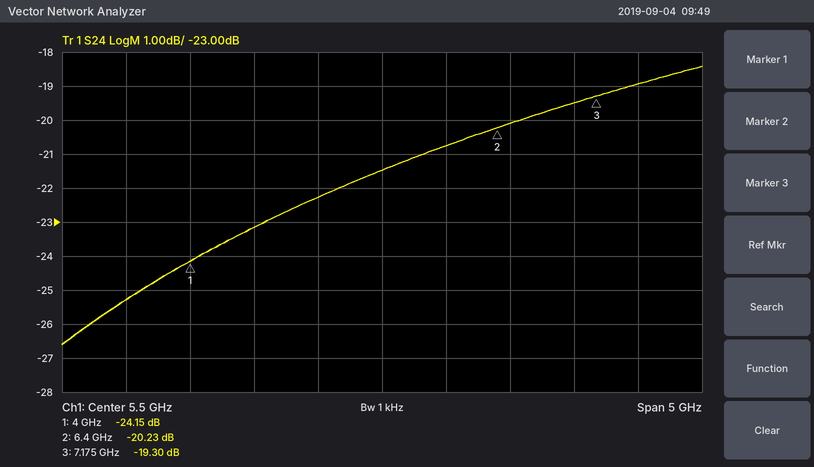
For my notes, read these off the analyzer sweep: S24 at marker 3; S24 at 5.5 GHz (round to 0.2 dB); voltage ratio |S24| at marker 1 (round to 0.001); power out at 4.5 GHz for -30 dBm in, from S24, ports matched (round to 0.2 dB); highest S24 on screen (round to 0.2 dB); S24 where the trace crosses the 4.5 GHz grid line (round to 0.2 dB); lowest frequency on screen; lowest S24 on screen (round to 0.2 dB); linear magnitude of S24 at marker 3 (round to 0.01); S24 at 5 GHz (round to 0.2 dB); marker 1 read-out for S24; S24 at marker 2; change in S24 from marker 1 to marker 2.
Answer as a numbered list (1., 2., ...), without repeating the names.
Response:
1. -19.30 dB
2. -21.4 dB
3. 0.062
4. -53.2 dBm
5. -18.4 dB
6. -23.2 dB
7. 3 GHz
8. -26.6 dB
9. 0.11
10. -22.2 dB
11. -24.15 dB
12. -20.23 dB
13. 3.92 dB
